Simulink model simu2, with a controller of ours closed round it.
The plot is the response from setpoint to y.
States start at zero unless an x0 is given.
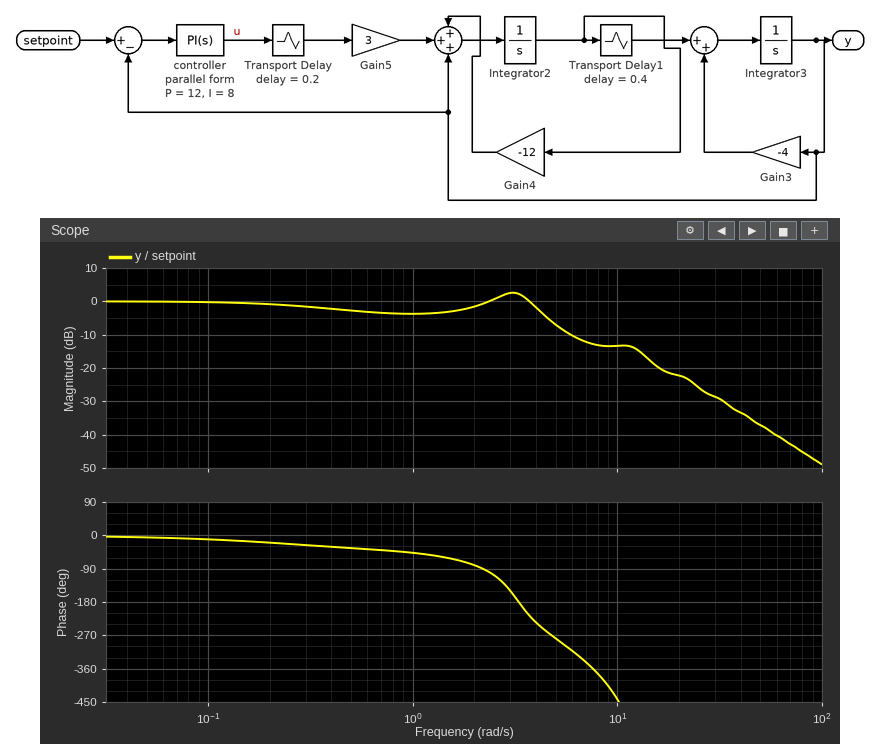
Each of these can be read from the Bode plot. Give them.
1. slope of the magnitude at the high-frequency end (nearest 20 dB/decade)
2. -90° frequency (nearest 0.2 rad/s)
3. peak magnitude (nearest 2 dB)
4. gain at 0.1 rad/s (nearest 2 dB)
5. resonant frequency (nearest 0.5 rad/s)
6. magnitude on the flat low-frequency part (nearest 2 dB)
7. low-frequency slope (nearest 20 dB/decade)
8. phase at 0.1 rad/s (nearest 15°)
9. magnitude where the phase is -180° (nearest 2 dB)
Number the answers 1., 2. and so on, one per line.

1. -40 dB/decade
2. 2.2 rad/s
3. 2 dB
4. 0 dB
5. 3.0 rad/s
6. 0 dB
7. 0 dB/decade
8. -15°
9. 2 dB
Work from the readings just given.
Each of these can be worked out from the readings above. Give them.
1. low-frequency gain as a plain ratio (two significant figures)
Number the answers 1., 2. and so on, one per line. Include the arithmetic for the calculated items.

1. 10^(0 / 20) = 1.0
